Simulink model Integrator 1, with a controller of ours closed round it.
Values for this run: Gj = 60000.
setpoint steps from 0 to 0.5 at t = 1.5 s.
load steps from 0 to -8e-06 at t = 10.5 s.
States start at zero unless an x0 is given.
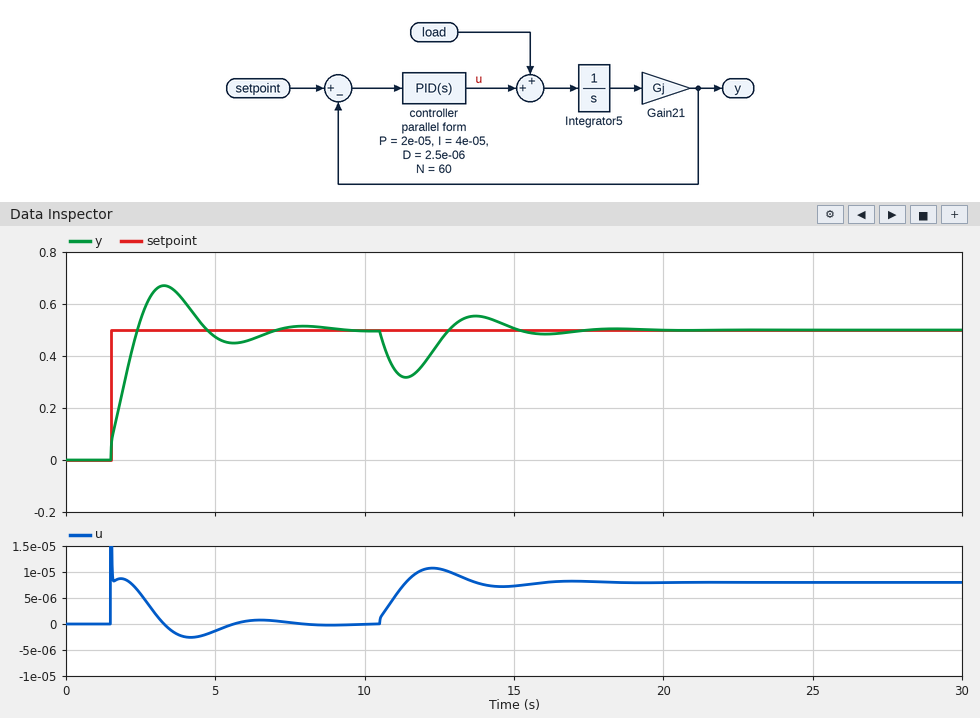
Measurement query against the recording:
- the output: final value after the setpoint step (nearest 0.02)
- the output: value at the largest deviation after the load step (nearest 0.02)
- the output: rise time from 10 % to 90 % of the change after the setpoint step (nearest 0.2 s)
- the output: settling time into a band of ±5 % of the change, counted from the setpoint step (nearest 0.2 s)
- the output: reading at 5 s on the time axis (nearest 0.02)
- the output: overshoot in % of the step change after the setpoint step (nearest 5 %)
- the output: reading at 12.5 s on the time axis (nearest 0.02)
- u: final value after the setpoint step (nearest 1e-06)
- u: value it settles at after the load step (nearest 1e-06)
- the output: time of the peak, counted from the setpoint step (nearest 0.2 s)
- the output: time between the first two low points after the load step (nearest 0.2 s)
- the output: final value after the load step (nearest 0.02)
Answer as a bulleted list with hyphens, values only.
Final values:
- 0.50
- 0.32
- 0.8 s
- 5.0 s
- 0.48
- 35 %
- 0.46
- 0.000000
- 0.000008
- 1.8 s
- 4.6 s
- 0.50
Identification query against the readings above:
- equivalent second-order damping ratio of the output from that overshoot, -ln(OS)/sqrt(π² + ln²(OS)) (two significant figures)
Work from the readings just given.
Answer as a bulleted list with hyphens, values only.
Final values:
- 0.32
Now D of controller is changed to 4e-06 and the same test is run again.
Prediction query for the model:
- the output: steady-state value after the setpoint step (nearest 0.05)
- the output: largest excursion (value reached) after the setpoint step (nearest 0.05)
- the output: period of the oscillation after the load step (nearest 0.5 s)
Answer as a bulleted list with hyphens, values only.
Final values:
- 0.50
- 0.65
- 5.0 s
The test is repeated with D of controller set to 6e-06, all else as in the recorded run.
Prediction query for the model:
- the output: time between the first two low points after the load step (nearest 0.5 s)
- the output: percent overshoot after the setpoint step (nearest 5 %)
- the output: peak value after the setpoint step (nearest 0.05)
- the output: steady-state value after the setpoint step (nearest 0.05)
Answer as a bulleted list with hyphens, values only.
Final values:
- 5.0 s
- 30 %
- 0.65
- 0.50
